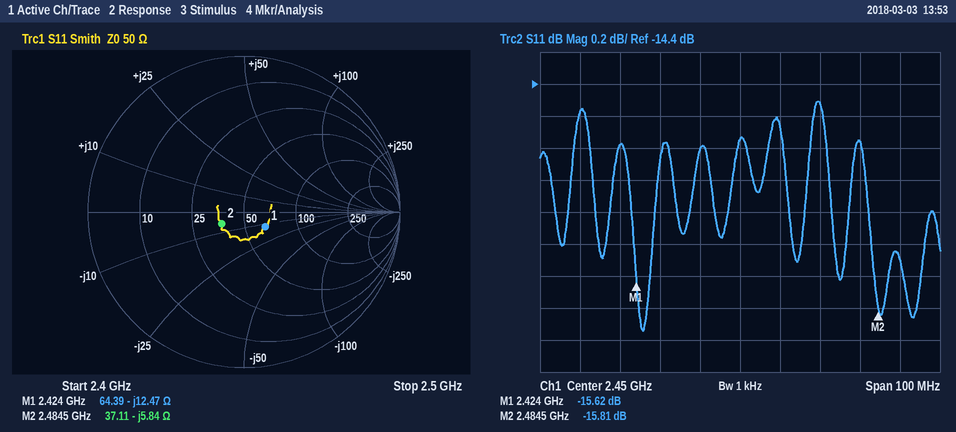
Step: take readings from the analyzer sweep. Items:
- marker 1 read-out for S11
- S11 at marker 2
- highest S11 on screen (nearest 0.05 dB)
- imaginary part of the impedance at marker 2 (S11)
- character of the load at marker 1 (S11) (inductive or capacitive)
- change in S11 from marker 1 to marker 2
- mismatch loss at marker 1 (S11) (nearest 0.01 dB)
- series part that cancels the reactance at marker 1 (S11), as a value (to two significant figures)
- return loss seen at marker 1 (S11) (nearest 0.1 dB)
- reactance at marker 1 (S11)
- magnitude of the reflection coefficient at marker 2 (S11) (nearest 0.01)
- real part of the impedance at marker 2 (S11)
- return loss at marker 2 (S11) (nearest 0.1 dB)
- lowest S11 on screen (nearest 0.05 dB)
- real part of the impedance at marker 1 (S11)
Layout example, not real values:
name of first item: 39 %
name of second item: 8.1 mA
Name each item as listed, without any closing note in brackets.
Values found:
marker 1 read-out for S11: -15.62 dB
S11 at marker 2: -15.81 dB
highest S11 on screen: -14.50 dB
imaginary part of the impedance at marker 2: -5.84 Ω
character of the load at marker 1 (S11): capacitive
change in S11 from marker 1 to marker 2: -0.19 dB
mismatch loss at marker 1 (S11): 0.12 dB
series part that cancels the reactance at marker 1 (S11), as a value: 820 pH
return loss seen at marker 1 (S11): 15.6 dB
reactance at marker 1: -12.47 Ω
magnitude of the reflection coefficient at marker 2 (S11): 0.16
real part of the impedance at marker 2: 37.11 Ω
return loss at marker 2 (S11): 15.8 dB
lowest S11 on screen: -15.95 dB
real part of the impedance at marker 1: 64.39 Ω
